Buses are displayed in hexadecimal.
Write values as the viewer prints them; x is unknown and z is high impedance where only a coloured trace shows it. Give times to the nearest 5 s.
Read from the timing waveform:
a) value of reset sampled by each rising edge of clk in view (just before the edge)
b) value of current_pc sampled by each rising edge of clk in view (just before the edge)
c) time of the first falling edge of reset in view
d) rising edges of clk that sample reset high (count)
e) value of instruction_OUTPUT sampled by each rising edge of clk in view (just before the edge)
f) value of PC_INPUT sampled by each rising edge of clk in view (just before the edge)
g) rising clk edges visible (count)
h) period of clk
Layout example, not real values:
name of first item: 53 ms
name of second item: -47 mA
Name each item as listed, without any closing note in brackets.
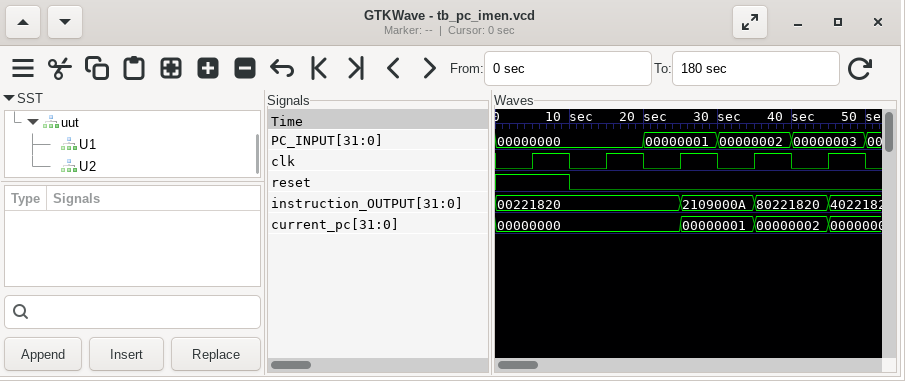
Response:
value of reset sampled by each rising edge of clk in view: 1 0 0 0 0
value of current_pc sampled by each rising edge of clk in view: 00000000, 00000000, 00000000, 00000001, 00000002
time of the first falling edge of reset in view: 10 s
rising edges of clk that sample reset high: 1
value of instruction_OUTPUT sampled by each rising edge of clk in view: 00221820, 00221820, 00221820, 2109000A, 80221820
value of PC_INPUT sampled by each rising edge of clk in view: 00000000, 00000000, 00000001, 00000002, 00000003
rising clk edges visible: 5
period of clk: 10 s
